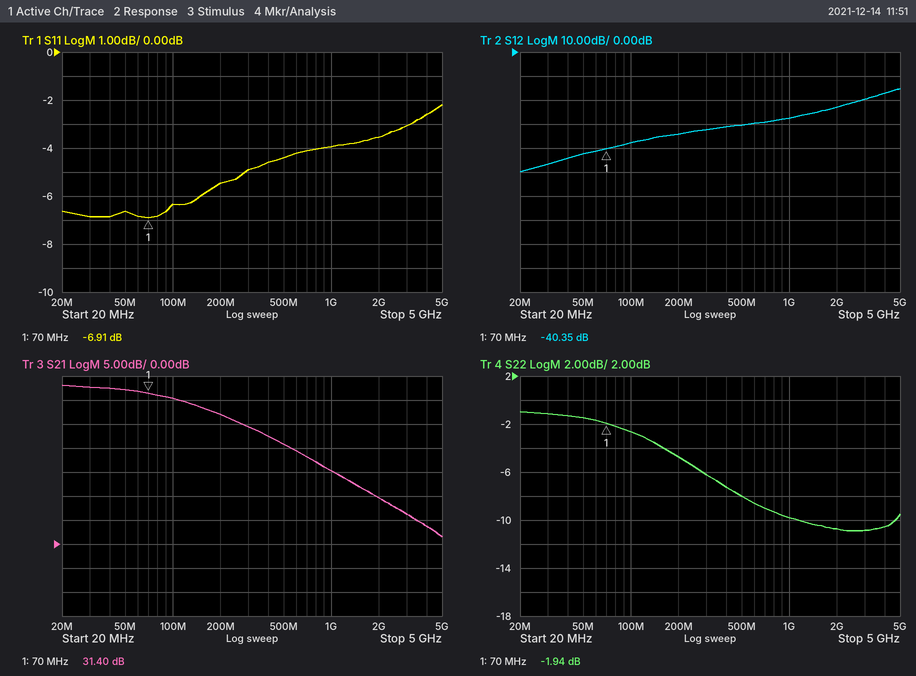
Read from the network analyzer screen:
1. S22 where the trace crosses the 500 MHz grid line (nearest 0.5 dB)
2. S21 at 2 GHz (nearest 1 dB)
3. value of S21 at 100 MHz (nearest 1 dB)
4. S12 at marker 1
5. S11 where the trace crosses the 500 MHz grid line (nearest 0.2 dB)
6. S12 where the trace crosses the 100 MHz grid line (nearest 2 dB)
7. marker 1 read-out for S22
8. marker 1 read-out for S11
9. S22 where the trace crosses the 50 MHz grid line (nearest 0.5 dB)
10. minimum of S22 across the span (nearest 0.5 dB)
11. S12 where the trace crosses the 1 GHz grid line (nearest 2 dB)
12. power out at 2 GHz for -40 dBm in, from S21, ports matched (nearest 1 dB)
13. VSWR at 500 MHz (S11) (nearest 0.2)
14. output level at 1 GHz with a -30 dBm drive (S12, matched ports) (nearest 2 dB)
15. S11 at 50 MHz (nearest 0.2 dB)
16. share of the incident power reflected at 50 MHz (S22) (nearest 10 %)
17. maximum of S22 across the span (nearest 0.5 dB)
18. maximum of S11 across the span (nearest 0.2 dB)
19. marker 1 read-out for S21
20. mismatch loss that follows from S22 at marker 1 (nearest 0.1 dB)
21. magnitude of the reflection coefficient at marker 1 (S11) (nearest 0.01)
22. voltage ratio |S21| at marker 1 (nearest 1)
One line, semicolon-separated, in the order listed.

-8.0 dB; 10 dB; 30 dB; -40.35 dB; -4.4 dB; -38 dB; -1.94 dB; -6.91 dB; -1.5 dB; -11.0 dB; -28 dB; -30 dBm; 4.0; -58 dBm; -6.6 dB; 70 %; -1.0 dB; -2.2 dB; 31.40 dB; 4.4 dB; 0.45; 37
